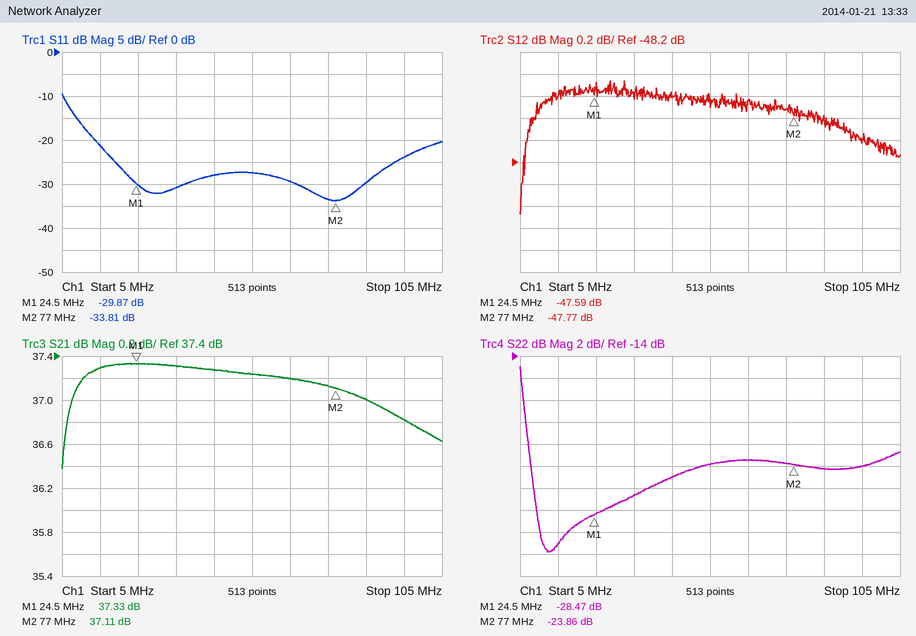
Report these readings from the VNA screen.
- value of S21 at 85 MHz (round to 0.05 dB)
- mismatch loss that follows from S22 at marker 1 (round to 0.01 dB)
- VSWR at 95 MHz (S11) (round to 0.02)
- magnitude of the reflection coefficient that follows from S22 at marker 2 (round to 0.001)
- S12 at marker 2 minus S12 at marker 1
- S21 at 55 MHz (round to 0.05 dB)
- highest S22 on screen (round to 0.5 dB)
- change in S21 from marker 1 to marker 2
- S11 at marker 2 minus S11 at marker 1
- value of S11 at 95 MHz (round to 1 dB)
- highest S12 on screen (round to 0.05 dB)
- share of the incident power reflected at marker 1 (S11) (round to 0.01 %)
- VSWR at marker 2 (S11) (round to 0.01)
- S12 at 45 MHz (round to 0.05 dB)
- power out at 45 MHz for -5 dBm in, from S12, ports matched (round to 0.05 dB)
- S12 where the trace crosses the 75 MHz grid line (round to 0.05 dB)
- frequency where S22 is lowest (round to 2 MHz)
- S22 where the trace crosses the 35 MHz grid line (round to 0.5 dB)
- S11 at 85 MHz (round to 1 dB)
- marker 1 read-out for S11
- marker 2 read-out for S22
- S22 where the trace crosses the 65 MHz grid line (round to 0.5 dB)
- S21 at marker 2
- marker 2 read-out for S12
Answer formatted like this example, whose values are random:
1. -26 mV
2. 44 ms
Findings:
1. 37.00 dB
2. 0.01 dB
3. 1.14
4. 0.064
5. -0.18 dB
6. 37.25 dB
7. -15.0 dB
8. -0.22 dB
9. -3.94 dB
10. -24 dB
11. -47.45 dB
12. 0.10 %
13. 1.04
14. -47.60 dB
15. -52.60 dBm
16. -47.70 dB
17. 12 MHz
18. -26.5 dB
19. -30 dB
20. -29.87 dB
21. -23.86 dB
22. -23.5 dB
23. 37.11 dB
24. -47.77 dB
